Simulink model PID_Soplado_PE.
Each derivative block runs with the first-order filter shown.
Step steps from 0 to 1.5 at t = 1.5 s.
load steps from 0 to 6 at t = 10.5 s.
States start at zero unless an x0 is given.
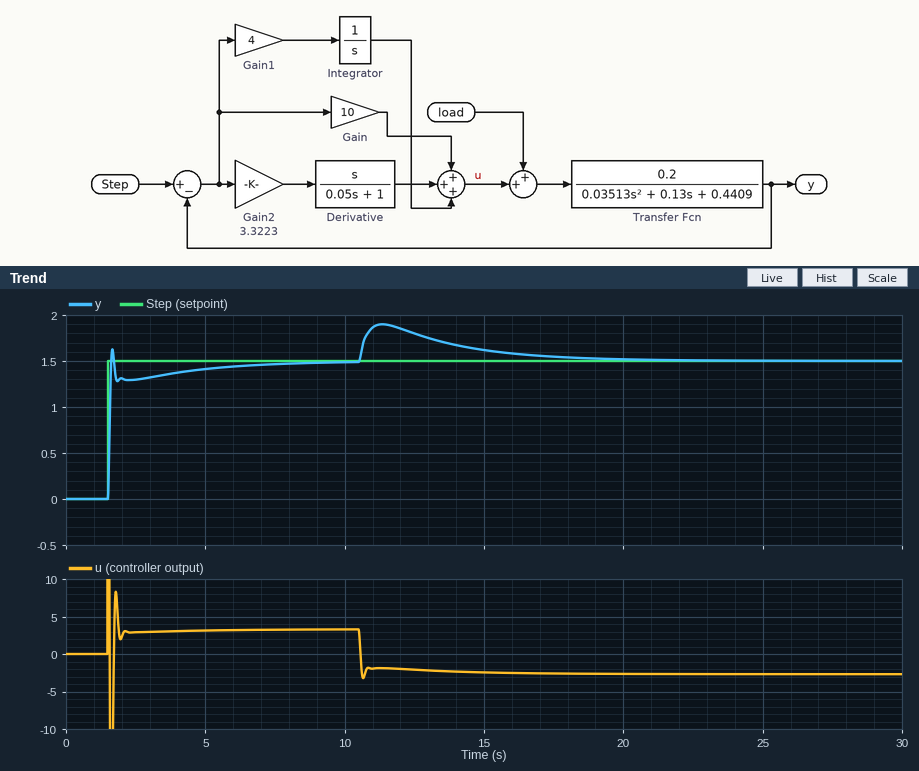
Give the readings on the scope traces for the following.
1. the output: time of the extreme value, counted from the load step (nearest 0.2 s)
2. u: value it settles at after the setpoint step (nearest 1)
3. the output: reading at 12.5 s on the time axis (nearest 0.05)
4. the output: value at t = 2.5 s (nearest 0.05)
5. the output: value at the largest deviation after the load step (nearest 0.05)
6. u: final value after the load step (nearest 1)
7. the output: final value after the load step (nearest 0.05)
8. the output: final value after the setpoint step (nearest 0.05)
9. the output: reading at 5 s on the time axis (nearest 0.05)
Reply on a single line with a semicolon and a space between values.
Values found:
0.8 s; 3; 1.80; 1.30; 1.90; -3; 1.50; 1.50; 1.40
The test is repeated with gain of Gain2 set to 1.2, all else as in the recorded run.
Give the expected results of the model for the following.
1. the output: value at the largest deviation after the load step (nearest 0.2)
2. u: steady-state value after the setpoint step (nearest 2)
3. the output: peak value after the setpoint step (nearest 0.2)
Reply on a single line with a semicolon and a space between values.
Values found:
2.0; 4; 1.6
